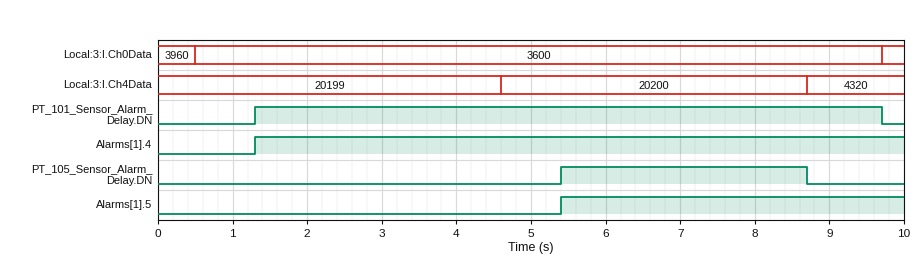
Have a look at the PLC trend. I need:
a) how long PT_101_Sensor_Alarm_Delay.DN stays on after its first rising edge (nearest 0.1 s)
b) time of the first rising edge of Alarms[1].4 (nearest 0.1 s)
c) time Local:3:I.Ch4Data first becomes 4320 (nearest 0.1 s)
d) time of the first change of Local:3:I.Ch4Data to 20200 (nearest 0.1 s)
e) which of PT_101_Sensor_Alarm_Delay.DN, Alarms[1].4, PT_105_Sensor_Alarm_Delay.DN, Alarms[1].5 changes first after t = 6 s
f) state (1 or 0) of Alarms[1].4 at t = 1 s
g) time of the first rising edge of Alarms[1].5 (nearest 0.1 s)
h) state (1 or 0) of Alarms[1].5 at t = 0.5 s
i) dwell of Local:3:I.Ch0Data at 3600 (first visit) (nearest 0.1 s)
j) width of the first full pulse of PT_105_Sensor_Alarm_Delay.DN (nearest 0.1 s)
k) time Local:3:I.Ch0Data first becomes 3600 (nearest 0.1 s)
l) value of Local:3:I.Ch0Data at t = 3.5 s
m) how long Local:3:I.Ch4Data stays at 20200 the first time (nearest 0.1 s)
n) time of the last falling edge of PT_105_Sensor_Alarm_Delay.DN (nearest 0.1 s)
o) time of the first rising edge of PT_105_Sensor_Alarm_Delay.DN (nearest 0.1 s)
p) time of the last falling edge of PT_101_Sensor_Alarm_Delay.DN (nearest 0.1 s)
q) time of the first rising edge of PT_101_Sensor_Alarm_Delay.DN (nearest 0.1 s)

8.4 s
1.3 s
8.7 s
4.6 s
PT_105_Sensor_Alarm_Delay.DN
0
5.4 s
0
9.2 s
3.3 s
0.5 s
3600
4.1 s
8.7 s
5.4 s
9.7 s
1.3 s
